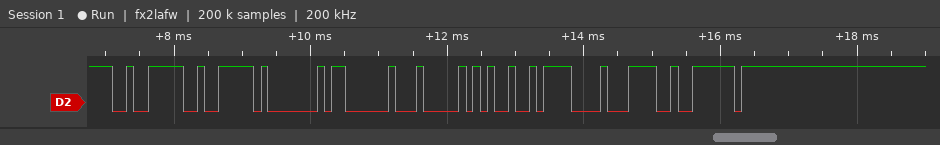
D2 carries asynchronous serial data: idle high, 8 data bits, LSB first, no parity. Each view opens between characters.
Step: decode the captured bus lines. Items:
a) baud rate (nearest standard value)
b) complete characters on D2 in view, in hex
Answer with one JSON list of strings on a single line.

["9600 baud", "F2, F2, 01, 03, 04, 25, 0F, 3C, 7E"]
